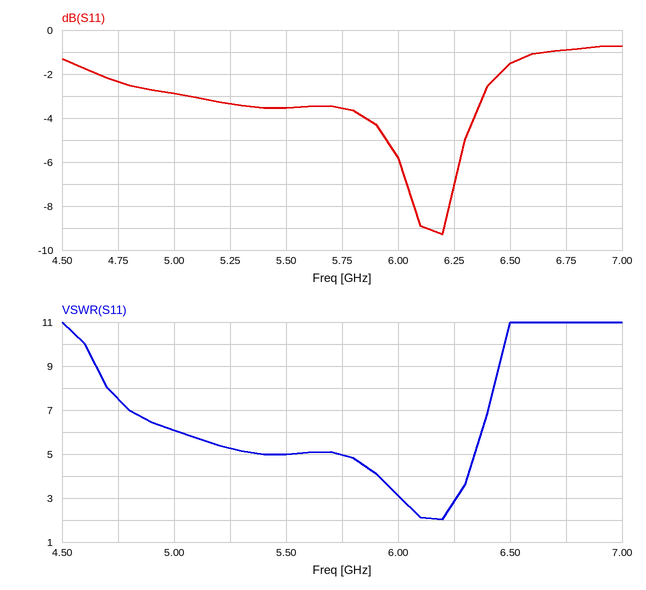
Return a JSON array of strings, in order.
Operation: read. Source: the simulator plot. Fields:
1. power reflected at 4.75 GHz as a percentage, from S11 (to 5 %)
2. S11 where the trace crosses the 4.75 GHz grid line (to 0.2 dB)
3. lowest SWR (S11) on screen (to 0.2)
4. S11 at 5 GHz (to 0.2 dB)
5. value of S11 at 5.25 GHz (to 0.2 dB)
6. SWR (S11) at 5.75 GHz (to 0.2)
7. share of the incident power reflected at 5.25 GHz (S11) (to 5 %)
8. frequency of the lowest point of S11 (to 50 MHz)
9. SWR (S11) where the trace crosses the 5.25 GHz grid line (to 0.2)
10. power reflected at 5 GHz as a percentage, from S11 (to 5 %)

["60 %", "-2.4 dB", "2.0", "-2.8 dB", "-3.4 dB", "5.0", "45 %", "6.20 GHz", "5.2", "50 %"]
